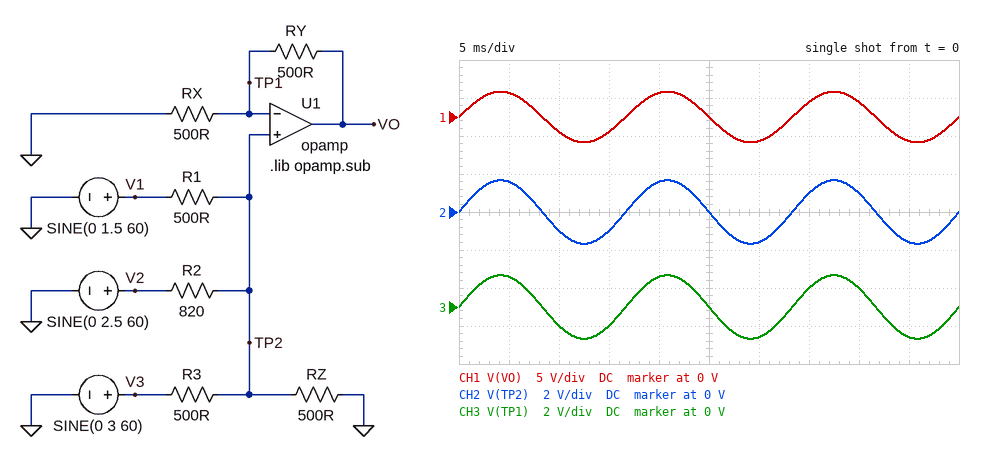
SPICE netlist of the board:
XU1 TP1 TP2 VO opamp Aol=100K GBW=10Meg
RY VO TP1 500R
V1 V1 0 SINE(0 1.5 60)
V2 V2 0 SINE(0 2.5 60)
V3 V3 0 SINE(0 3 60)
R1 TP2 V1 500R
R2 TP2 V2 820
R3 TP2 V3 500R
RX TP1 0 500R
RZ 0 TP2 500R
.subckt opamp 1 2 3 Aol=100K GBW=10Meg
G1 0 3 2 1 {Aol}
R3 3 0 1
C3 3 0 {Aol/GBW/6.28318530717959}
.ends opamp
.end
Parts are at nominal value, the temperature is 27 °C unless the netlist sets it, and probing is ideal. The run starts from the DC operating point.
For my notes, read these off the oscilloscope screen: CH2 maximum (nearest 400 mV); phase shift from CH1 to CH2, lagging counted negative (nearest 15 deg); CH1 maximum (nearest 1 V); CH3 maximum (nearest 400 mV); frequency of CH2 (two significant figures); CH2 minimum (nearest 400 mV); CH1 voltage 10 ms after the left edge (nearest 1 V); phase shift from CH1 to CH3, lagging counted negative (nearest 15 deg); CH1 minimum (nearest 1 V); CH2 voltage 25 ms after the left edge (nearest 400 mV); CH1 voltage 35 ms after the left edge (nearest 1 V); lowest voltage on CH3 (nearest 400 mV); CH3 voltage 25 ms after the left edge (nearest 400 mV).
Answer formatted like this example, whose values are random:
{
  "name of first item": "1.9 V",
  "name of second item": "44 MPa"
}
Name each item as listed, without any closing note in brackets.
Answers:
{
  "CH2 maximum": "1.6 V",
  "phase shift from CH1 to CH2, lagging counted negative": "0 deg",
  "CH1 maximum": "3 V",
  "CH3 maximum": "1.6 V",
  "frequency of CH2": "60 Hz",
  "CH2 minimum": "-1.6 V",
  "CH1 voltage 10 ms after the left edge": "-2 V",
  "phase shift from CH1 to CH3, lagging counted negative": "0 deg",
  "CH1 minimum": "-3 V",
  "CH2 voltage 25 ms after the left edge": "0 V",
  "CH1 voltage 35 ms after the left edge": "2 V",
  "lowest voltage on CH3": "-1.6 V",
  "CH3 voltage 25 ms after the left edge": "0 V"
}
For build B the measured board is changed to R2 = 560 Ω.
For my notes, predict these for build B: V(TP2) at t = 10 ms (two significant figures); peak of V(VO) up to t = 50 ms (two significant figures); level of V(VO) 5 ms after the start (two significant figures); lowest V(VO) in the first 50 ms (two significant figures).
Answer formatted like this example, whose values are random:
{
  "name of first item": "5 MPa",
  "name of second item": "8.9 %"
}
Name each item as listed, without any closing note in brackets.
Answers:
{
  "V(TP2) at t = 10 ms": "-1.0 V",
  "peak of V(VO) up to t = 50 ms": "3.5 V",
  "level of V(VO) 5 ms after the start": "3.3 V",
  "lowest V(VO) in the first 50 ms": "-3.5 V"
}
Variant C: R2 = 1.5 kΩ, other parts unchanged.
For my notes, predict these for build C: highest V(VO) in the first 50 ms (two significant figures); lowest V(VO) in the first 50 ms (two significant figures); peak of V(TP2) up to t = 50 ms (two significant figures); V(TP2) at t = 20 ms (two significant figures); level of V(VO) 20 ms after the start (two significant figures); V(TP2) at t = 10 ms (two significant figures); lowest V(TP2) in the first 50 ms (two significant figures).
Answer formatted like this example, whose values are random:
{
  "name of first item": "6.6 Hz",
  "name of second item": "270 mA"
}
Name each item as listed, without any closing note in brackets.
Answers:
{
  "highest V(VO) in the first 50 ms": "3.2 V",
  "lowest V(VO) in the first 50 ms": "-3.2 V",
  "peak of V(TP2) up to t = 50 ms": "1.6 V",
  "V(TP2) at t = 20 ms": "1.5 V",
  "level of V(VO) 20 ms after the start": "3.0 V",
  "V(TP2) at t = 10 ms": "-940 mV",
  "lowest V(TP2) in the first 50 ms": "-1.6 V"
}
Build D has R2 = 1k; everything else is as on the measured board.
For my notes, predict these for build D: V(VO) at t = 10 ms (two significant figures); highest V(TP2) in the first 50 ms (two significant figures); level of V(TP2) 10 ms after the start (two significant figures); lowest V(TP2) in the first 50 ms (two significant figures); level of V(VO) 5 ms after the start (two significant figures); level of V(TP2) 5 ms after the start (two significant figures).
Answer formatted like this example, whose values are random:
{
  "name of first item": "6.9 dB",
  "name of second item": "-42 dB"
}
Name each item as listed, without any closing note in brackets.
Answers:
{
  "V(VO) at t = 10 ms": "-1.9 V",
  "highest V(TP2) in the first 50 ms": "1.6 V",
  "level of V(TP2) 10 ms after the start": "-970 mV",
  "lowest V(TP2) in the first 50 ms": "-1.6 V",
  "level of V(VO) 5 ms after the start": "3.1 V",
  "level of V(TP2) 5 ms after the start": "1.6 V"
}
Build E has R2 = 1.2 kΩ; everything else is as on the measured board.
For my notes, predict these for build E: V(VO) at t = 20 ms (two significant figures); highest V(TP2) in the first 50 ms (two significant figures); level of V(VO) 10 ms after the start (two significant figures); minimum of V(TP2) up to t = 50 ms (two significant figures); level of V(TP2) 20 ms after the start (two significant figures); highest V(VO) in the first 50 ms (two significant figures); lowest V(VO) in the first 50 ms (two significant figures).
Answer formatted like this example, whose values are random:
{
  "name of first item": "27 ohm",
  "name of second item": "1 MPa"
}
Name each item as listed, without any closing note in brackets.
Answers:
{
  "V(VO) at t = 20 ms": "3.1 V",
  "highest V(TP2) in the first 50 ms": "1.6 V",
  "level of V(VO) 10 ms after the start": "-1.9 V",
  "minimum of V(TP2) up to t = 50 ms": "-1.6 V",
  "level of V(TP2) 20 ms after the start": "1.5 V",
  "highest V(VO) in the first 50 ms": "3.2 V",
  "lowest V(VO) in the first 50 ms": "-3.2 V"
}
